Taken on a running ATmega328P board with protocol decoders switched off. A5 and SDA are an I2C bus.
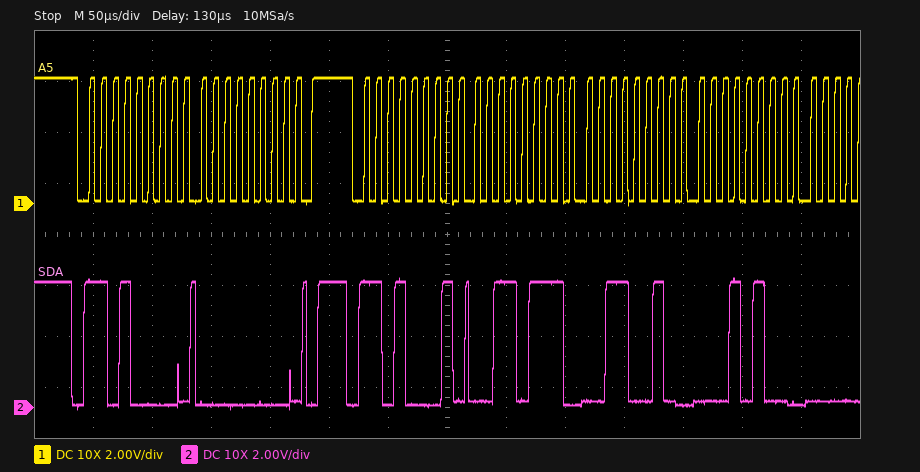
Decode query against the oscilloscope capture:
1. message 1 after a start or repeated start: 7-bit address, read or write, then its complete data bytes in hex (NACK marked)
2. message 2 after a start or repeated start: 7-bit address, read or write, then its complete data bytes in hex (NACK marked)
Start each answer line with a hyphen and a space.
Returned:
- 0x68 write: 00
- 0x68 read: 37 32 14
